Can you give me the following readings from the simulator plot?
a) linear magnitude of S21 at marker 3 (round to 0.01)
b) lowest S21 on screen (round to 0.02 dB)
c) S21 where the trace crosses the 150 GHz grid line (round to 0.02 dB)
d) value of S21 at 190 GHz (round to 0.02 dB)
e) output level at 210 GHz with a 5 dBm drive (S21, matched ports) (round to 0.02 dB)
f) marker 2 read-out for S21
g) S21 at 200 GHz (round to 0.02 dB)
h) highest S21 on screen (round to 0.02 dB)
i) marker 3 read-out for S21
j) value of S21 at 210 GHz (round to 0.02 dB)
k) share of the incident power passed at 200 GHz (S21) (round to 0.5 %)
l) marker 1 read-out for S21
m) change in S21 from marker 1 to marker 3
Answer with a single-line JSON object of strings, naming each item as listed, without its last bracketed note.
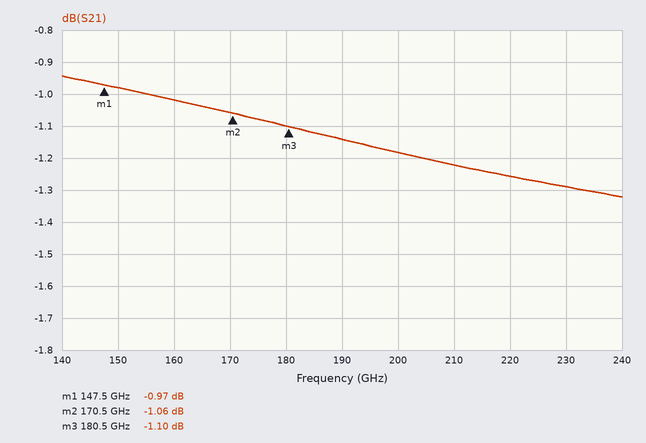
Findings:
{"linear magnitude of S21 at marker 3": "0.88", "lowest S21 on screen": "-1.32 dB", "S21 where the trace crosses the 150 GHz grid line": "-0.98 dB", "value of S21 at 190 GHz": "-1.14 dB", "output level at 210 GHz with a 5 dBm drive (S21, matched ports)": "3.78 dBm", "marker 2 read-out for S21": "-1.06 dB", "S21 at 200 GHz": "-1.18 dB", "highest S21 on screen": "-0.94 dB", "marker 3 read-out for S21": "-1.10 dB", "value of S21 at 210 GHz": "-1.22 dB", "share of the incident power passed at 200 GHz (S21)": "76.0 %", "marker 1 read-out for S21": "-0.97 dB", "change in S21 from marker 1 to marker 3": "-0.13 dB"}
